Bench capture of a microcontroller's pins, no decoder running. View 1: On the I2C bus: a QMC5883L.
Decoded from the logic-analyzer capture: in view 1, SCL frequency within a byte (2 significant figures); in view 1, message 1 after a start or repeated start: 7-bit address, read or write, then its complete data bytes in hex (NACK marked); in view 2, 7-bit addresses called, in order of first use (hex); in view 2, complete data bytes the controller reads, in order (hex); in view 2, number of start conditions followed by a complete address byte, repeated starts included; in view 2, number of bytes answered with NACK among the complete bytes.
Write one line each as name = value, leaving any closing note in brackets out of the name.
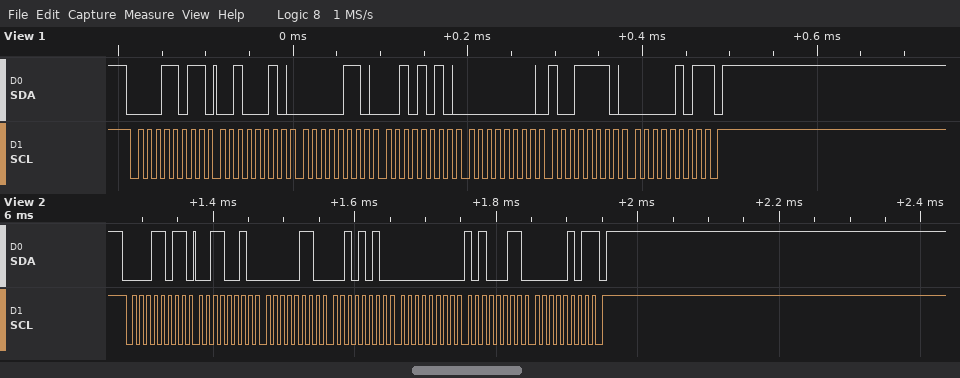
in view 1, SCL frequency within a byte = 100 kHz
in view 1, message 1 after a start or repeated start: 7-bit address, read or write, then its complete data bytes in hex = 0x0D read: 22 06 2A 00 9E 05 NACK
in view 2, 7-bit addresses called, in order of first use = 0x0D
in view 2, complete data bytes the controller reads, in order = 32 06 2A 00 A3 05
in view 2, number of start conditions followed by a complete address byte, repeated starts included = 1
in view 2, number of bytes answered with NACK among the complete bytes = 1
